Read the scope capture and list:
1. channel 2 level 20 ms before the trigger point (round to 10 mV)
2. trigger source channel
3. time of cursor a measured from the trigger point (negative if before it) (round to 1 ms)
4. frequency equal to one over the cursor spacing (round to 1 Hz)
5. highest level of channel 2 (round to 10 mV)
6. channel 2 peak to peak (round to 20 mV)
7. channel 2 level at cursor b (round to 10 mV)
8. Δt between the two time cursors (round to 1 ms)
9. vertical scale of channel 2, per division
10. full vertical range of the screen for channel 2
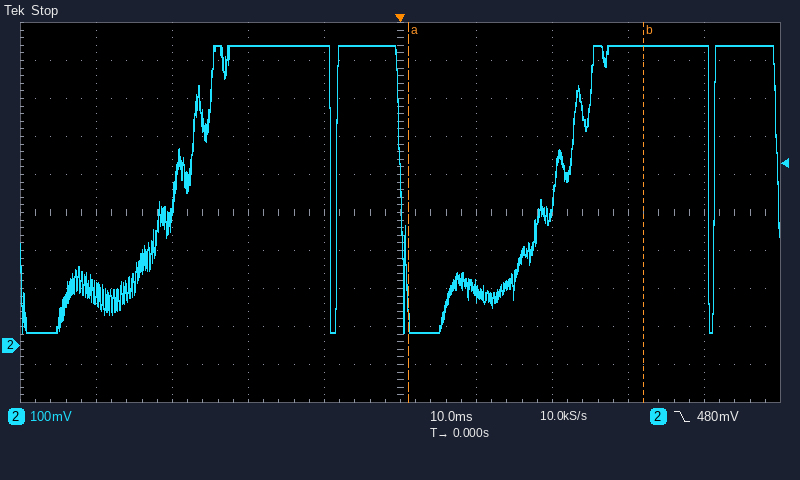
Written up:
790 mV
channel 2
+1 ms
32 Hz
790 mV
760 mV
790 mV
31 ms
100 mV
1 V
